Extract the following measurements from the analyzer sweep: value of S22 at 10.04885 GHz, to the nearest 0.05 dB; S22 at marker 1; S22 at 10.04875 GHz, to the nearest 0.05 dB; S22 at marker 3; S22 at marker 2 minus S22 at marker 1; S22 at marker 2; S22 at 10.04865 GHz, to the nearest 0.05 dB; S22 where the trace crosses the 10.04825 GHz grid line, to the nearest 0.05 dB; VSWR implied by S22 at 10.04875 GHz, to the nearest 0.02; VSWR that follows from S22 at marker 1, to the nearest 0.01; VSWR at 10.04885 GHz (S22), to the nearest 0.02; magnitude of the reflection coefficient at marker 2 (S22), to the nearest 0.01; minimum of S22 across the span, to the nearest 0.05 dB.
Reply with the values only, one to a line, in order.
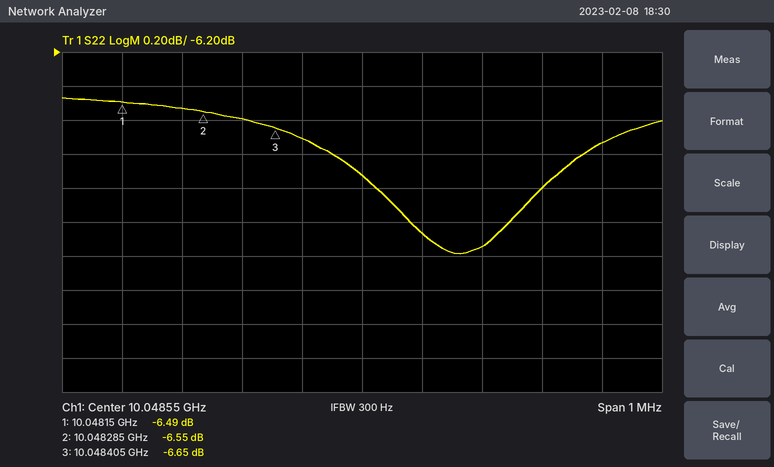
-7.00 dB
-6.49 dB
-7.35 dB
-6.65 dB
-0.06 dB
-6.55 dB
-7.25 dB
-6.55 dB
2.50
2.80
2.62
0.47
-7.40 dB
